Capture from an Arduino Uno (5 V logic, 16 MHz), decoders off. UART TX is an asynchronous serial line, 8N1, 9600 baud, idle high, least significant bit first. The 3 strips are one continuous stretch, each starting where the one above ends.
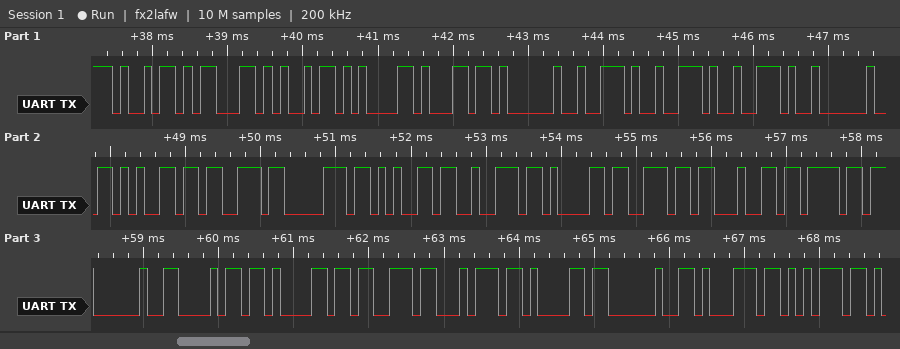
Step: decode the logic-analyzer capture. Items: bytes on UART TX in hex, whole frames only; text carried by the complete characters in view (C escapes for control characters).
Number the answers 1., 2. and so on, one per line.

1. 69 63 69 61 6C 20 2E 2E 2E 20 65 73 70 65 72 61 6E 64 6F 20 68 61 73 74 61 20 71 75
2. "icial ... esperando hasta qu"
